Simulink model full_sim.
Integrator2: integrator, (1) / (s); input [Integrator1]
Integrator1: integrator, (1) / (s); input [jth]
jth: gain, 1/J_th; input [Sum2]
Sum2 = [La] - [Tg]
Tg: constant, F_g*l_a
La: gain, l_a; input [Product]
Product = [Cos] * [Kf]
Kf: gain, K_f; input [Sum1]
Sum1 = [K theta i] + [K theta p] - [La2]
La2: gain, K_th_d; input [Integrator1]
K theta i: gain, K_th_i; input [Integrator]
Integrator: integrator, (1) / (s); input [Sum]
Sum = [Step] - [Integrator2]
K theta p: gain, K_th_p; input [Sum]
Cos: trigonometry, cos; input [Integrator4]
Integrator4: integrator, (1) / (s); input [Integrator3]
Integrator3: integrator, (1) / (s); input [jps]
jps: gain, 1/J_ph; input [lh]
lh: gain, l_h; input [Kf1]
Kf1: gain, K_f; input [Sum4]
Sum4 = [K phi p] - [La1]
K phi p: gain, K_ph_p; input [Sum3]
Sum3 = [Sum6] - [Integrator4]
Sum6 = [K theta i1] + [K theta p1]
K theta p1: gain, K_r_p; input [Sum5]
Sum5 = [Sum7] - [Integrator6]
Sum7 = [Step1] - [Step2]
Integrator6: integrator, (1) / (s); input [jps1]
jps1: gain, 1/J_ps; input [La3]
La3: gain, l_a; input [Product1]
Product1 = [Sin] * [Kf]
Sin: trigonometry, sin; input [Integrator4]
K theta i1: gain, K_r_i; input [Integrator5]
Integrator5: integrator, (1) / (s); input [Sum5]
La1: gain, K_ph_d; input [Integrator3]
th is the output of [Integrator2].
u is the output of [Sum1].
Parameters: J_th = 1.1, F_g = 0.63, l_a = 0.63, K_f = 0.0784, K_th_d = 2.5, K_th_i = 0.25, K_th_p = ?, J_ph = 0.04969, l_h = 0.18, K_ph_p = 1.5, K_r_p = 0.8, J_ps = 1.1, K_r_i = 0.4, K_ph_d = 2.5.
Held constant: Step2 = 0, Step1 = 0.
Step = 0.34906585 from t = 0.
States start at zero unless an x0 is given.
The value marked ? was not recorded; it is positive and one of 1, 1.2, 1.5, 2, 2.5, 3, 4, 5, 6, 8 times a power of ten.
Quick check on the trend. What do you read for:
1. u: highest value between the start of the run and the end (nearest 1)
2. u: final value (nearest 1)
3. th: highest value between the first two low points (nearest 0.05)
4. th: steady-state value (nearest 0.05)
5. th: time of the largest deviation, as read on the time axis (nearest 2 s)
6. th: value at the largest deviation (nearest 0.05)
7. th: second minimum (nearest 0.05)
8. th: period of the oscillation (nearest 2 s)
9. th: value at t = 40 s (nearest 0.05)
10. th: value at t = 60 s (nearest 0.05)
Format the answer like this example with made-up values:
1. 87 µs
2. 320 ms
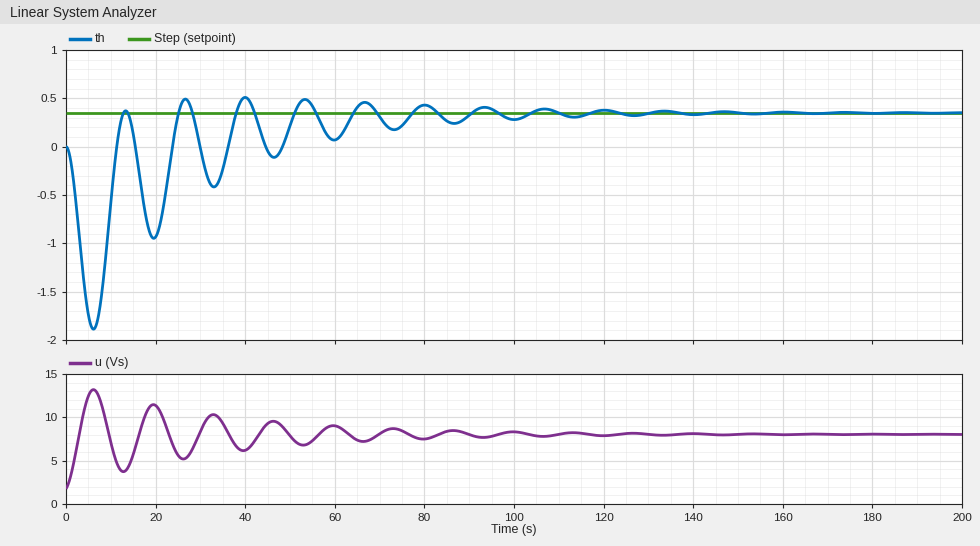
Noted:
1. 13
2. 8
3. 0.35
4. 0.35
5. 6 s
6. -1.90
7. -0.95
8. 14 s
9. 0.50
10. 0.05
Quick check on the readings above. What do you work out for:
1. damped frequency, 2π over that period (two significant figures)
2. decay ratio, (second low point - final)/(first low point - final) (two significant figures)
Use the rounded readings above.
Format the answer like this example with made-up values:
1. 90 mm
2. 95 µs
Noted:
1. 0.45 rad/s
2. 0.58
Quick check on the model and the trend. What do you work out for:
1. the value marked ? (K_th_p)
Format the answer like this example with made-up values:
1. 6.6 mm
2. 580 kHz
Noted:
1. 5
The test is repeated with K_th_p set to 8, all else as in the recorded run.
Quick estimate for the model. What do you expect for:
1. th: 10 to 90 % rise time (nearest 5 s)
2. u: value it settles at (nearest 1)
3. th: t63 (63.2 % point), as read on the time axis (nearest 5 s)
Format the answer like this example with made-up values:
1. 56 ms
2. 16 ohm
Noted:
1. 95 s
2. 8
3. 50 s
